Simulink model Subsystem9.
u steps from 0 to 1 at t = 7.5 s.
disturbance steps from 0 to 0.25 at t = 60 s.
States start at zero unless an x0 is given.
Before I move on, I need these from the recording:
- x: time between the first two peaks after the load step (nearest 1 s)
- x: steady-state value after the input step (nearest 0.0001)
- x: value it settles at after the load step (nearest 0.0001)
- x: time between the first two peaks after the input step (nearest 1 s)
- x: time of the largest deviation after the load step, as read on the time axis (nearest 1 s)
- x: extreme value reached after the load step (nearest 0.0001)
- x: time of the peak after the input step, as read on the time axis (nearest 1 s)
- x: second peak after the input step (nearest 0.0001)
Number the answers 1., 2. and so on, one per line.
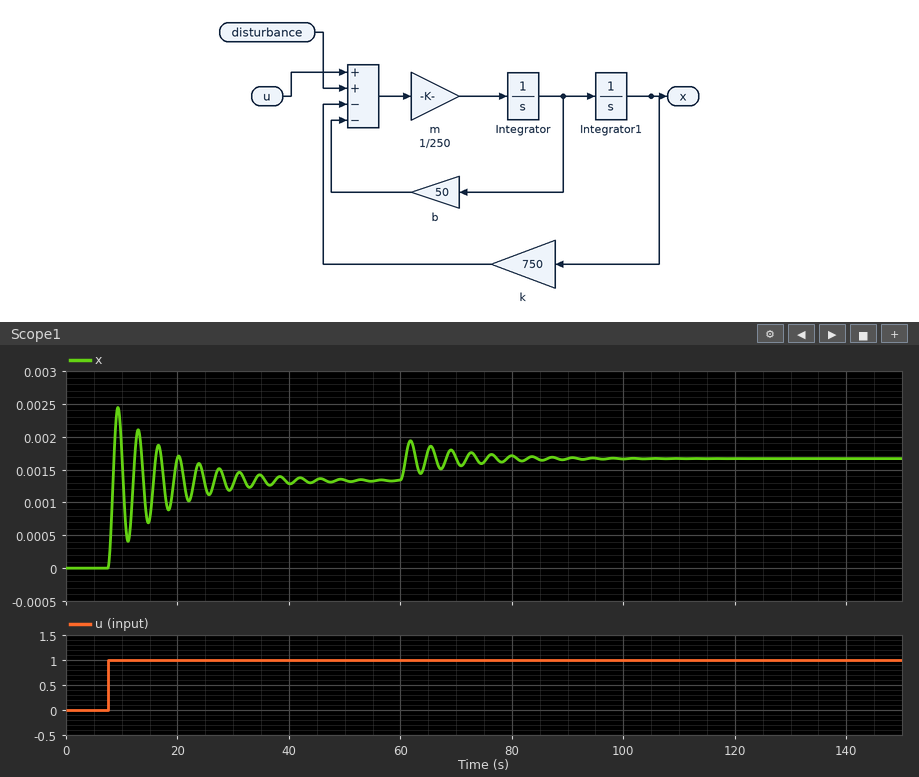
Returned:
1. 4 s
2. 0.0013
3. 0.0017
4. 4 s
5. 62 s
6. 0.0019
7. 9 s
8. 0.0021
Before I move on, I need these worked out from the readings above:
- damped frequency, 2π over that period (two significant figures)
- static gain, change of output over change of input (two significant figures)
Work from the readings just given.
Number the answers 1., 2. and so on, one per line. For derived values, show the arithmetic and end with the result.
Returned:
1. 2π / 4 = 1.6 rad/s
2. (0.0013 - 0) / (1 - 0) = 0.0013
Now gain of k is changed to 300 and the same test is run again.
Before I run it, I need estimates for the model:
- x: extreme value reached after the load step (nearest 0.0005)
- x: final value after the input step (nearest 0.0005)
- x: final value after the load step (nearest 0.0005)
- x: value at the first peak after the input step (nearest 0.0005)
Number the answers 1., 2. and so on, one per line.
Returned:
1. 0.0050
2. 0.0035
3. 0.0040
4. 0.0060
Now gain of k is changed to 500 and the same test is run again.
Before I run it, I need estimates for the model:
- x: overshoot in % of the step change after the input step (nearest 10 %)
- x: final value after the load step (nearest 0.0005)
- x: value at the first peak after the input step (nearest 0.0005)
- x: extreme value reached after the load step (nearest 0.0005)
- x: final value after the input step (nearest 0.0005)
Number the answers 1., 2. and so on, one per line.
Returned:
1. 80 %
2. 0.0025
3. 0.0035
4. 0.0030
5. 0.0020
